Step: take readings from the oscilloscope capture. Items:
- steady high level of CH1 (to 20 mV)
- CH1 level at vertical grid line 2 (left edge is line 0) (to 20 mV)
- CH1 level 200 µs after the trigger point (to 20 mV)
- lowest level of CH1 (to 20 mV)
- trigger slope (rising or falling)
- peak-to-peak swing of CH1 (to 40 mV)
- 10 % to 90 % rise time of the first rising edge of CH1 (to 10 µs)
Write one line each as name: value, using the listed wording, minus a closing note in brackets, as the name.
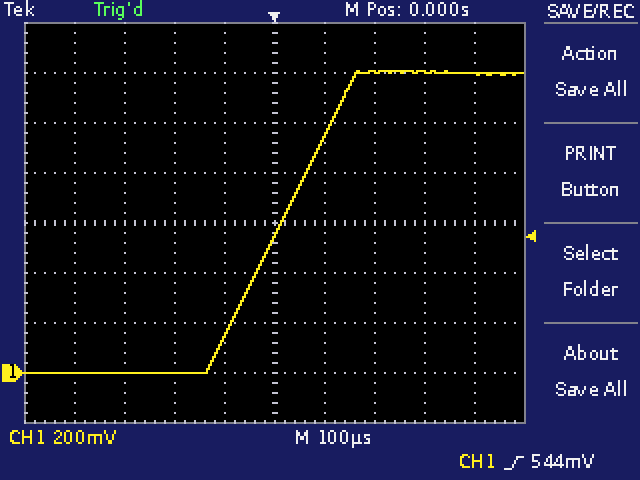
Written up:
steady high level of CH1: 1.20 V
CH1 level at vertical grid line 2 (left edge is line 0): 0 mV
CH1 level 200 µs after the trigger point: 1.20 V
lowest level of CH1: 0 mV
trigger slope: rising
peak-to-peak swing of CH1: 1.20 V
10 % to 90 % rise time of the first rising edge of CH1: 240 µs
